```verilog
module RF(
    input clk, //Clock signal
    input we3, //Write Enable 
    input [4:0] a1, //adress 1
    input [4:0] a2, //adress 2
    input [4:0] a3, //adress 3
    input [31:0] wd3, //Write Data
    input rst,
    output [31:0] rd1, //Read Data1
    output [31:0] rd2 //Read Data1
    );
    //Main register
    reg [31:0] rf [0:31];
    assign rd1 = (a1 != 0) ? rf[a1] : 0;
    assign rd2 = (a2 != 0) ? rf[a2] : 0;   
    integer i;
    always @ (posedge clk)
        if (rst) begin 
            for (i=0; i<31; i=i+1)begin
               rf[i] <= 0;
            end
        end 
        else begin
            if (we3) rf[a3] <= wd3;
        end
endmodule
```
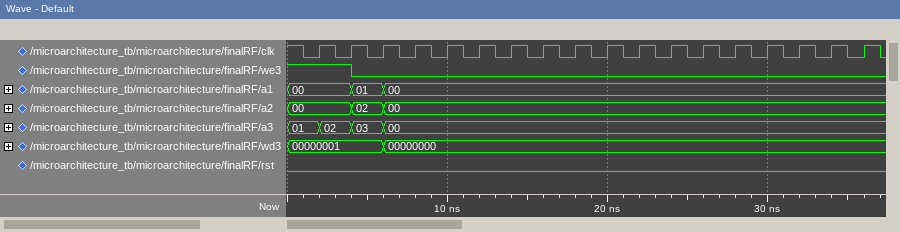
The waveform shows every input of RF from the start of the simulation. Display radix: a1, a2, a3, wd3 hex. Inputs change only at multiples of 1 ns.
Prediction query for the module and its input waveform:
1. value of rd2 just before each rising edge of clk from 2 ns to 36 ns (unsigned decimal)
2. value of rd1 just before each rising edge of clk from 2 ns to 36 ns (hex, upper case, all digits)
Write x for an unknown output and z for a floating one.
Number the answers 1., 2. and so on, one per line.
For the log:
1. 0, 0, 1, 0, 0, 0, 0, 0, 0, 0, 0, 0, 0, 0, 0, 0, 0, 0
2. 00000000, 00000000, 00000001, 00000000, 00000000, 00000000, 00000000, 00000000, 00000000, 00000000, 00000000, 00000000, 00000000, 00000000, 00000000, 00000000, 00000000, 00000000
